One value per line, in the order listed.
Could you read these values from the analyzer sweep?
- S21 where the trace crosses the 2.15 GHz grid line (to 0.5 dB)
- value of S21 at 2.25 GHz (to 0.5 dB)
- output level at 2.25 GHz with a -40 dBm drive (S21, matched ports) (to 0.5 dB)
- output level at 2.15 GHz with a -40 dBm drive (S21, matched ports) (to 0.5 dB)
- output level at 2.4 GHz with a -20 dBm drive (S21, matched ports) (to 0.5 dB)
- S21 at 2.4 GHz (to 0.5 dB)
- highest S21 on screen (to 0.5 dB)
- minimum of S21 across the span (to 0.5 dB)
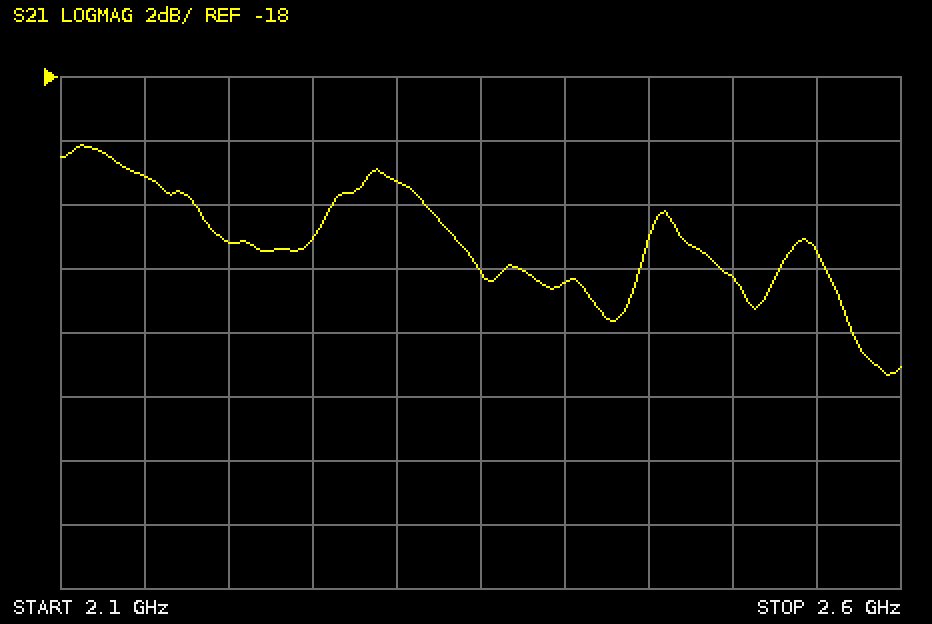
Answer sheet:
-21.0 dB
-23.0 dB
-63.0 dBm
-61.0 dBm
-44.5 dBm
-24.5 dB
-20.0 dB
-27.5 dB
